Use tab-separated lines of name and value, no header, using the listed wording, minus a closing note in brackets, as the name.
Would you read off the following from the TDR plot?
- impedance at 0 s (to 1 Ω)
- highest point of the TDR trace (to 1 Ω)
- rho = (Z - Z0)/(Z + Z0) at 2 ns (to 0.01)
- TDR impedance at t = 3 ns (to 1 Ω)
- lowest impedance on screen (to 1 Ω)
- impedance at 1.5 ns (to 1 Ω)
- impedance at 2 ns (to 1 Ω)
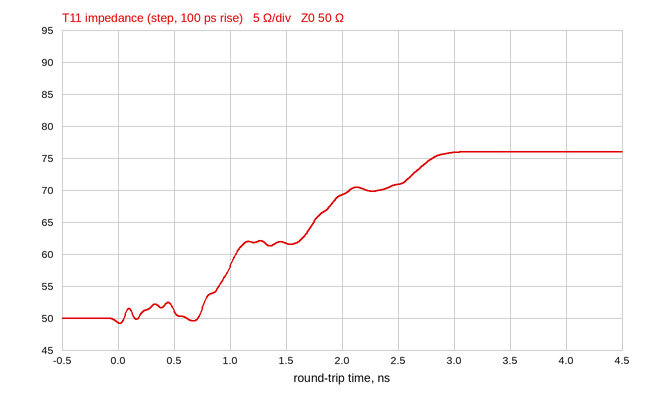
impedance at 0 s	49 Ω
highest point of the TDR trace	76 Ω
rho = (Z - Z0)/(Z + Z0) at 2 ns	+0.16
TDR impedance at t = 3 ns	76 Ω
lowest impedance on screen	49 Ω
impedance at 1.5 ns	62 Ω
impedance at 2 ns	69 Ω
